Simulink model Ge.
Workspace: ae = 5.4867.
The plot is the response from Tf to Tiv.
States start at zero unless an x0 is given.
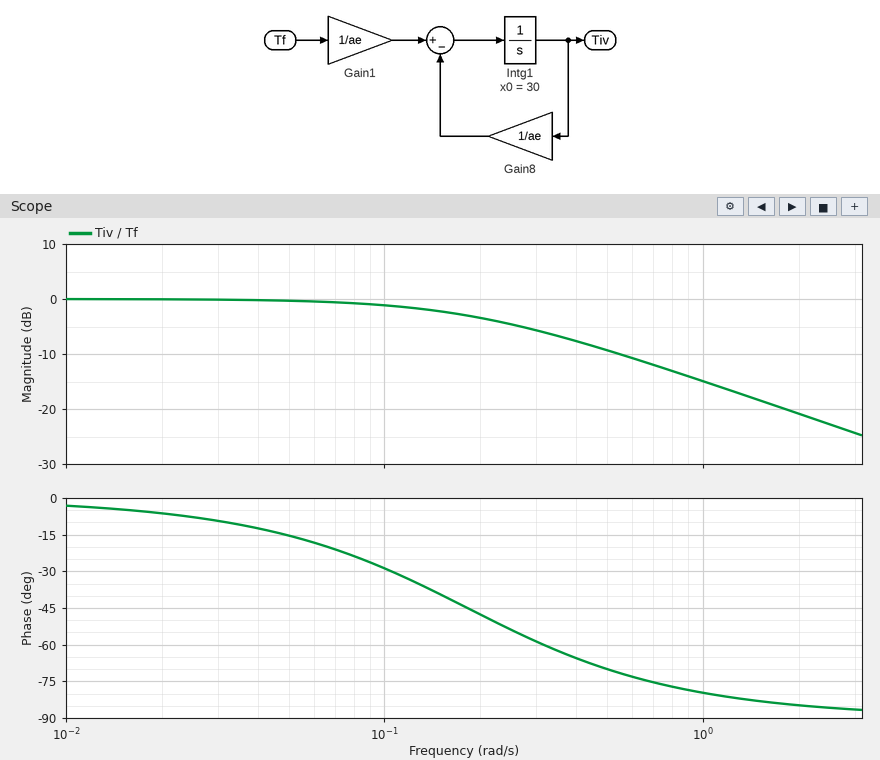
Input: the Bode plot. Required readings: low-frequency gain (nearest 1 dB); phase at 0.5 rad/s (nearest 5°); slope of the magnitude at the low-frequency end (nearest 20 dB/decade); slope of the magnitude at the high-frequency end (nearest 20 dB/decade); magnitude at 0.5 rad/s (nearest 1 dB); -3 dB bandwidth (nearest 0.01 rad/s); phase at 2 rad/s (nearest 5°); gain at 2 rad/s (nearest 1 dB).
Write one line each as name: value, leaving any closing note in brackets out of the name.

low-frequency gain: 0 dB
phase at 0.5 rad/s: -70°
slope of the magnitude at the low-frequency end: 0 dB/decade
slope of the magnitude at the high-frequency end: -20 dB/decade
magnitude at 0.5 rad/s: -9 dB
-3 dB bandwidth: 0.18 rad/s
phase at 2 rad/s: -85°
gain at 2 rad/s: -21 dB
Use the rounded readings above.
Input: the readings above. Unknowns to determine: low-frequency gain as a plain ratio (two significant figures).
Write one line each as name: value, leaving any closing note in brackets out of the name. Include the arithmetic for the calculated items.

low-frequency gain as a plain ratio: 10^(0 / 20) = 1.0
